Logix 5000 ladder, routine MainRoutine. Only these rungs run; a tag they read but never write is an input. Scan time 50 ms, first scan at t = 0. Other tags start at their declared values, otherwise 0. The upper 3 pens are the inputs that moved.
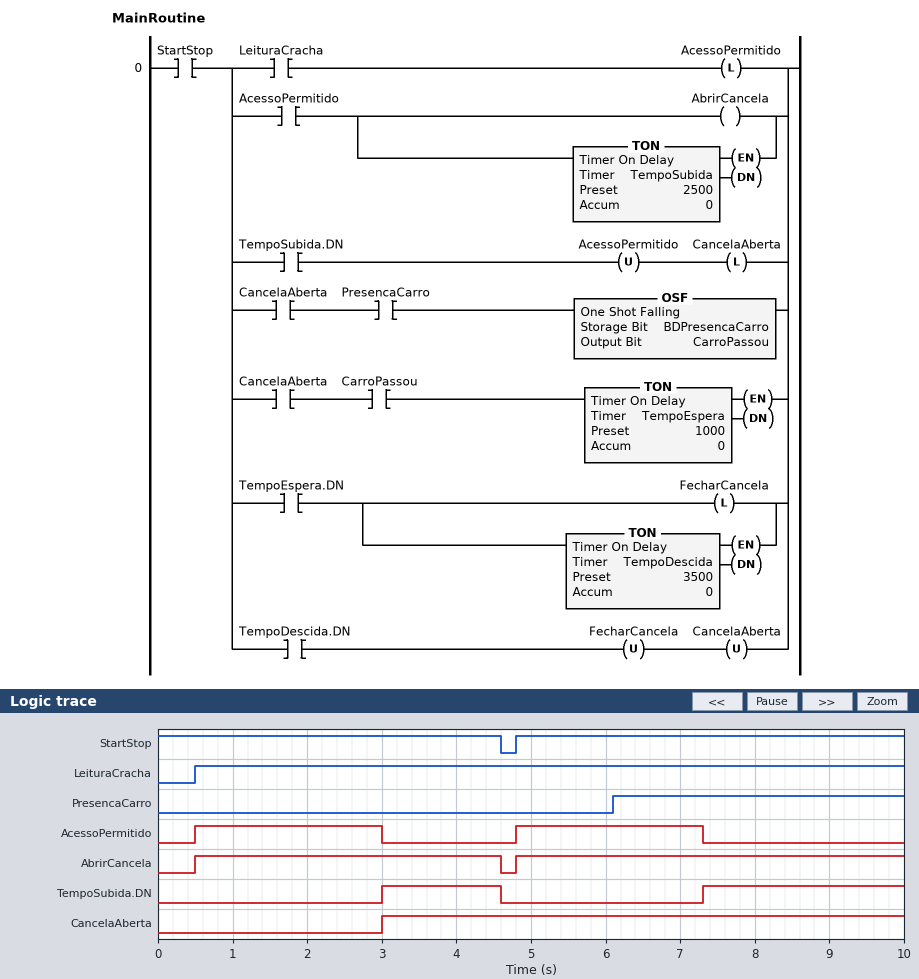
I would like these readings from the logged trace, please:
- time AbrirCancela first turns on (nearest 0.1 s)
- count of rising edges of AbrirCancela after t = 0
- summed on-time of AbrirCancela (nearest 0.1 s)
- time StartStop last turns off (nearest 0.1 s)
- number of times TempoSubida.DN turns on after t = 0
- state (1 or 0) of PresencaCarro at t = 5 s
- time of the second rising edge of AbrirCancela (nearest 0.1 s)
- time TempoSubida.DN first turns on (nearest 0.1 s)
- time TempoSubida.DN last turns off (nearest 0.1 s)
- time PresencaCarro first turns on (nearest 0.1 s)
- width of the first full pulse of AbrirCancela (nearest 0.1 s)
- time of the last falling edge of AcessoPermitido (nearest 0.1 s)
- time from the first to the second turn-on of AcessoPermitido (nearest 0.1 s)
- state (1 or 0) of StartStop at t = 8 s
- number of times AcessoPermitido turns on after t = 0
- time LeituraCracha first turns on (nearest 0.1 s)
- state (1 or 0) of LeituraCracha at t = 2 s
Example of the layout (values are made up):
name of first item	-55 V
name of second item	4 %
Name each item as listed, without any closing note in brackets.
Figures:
time AbrirCancela first turns on	0.5 s
count of rising edges of AbrirCancela after t = 0	2
summed on-time of AbrirCancela	9.3 s
time StartStop last turns off	4.6 s
number of times TempoSubida.DN turns on after t = 0	2
state (1 or 0) of PresencaCarro at t = 5 s	0
time of the second rising edge of AbrirCancela	4.8 s
time TempoSubida.DN first turns on	3.0 s
time TempoSubida.DN last turns off	4.6 s
time PresencaCarro first turns on	6.1 s
width of the first full pulse of AbrirCancela	4.1 s
time of the last falling edge of AcessoPermitido	7.3 s
time from the first to the second turn-on of AcessoPermitido	4.3 s
state (1 or 0) of StartStop at t = 8 s	1
number of times AcessoPermitido turns on after t = 0	2
time LeituraCracha first turns on	0.5 s
state (1 or 0) of LeituraCracha at t = 2 s	1
